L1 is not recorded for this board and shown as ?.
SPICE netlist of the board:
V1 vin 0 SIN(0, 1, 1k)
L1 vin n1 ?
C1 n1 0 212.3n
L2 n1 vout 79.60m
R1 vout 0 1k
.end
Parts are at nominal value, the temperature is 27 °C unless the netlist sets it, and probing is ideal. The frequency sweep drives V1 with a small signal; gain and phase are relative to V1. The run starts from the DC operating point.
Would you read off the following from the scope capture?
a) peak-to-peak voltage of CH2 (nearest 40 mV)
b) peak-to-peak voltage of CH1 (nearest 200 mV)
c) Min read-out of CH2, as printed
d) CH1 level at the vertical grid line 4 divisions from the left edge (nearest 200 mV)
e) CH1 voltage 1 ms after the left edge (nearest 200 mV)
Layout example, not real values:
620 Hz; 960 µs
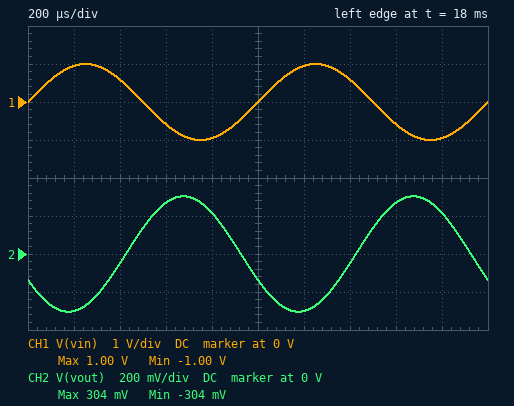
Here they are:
600 mV; 2.0 V; -304 mV; -1.0 V; 0 V
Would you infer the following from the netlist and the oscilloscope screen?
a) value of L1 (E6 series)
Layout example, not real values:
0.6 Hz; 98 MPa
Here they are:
470 mH
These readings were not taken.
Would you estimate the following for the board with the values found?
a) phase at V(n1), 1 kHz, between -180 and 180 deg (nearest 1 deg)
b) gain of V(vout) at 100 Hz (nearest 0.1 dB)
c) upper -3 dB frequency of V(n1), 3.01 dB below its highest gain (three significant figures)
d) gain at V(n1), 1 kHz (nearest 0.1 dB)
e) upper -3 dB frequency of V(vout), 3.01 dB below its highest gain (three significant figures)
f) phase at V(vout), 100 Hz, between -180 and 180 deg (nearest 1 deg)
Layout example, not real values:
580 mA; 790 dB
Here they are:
-127 deg; -0.2 dB; 487 Hz; -9.4 dB; 464 Hz; -20 deg
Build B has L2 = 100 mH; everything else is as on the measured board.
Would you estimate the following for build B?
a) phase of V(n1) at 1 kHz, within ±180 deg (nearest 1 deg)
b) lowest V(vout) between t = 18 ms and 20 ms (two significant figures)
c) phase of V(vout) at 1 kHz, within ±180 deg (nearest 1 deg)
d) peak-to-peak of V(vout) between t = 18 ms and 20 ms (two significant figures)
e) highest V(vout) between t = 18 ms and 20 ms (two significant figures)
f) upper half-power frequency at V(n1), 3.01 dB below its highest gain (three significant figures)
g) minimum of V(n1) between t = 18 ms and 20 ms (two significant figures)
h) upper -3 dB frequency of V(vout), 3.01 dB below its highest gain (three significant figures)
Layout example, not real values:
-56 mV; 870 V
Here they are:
-127 deg; -320 mV; -159 deg; 640 mV; 320 mV; 501 Hz; -380 mV; 459 Hz
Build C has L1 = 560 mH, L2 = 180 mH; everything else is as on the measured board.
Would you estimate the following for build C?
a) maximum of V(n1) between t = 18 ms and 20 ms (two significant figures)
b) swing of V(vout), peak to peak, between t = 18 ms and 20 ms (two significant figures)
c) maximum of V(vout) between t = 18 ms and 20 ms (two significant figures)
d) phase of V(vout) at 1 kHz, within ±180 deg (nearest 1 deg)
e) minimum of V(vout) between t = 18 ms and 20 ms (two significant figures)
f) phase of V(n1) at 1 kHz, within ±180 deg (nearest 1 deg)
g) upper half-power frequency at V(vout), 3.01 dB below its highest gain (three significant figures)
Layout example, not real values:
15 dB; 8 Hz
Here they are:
400 mV; 530 mV; 270 mV; 170 deg; -270 mV; -142 deg; 321 Hz
